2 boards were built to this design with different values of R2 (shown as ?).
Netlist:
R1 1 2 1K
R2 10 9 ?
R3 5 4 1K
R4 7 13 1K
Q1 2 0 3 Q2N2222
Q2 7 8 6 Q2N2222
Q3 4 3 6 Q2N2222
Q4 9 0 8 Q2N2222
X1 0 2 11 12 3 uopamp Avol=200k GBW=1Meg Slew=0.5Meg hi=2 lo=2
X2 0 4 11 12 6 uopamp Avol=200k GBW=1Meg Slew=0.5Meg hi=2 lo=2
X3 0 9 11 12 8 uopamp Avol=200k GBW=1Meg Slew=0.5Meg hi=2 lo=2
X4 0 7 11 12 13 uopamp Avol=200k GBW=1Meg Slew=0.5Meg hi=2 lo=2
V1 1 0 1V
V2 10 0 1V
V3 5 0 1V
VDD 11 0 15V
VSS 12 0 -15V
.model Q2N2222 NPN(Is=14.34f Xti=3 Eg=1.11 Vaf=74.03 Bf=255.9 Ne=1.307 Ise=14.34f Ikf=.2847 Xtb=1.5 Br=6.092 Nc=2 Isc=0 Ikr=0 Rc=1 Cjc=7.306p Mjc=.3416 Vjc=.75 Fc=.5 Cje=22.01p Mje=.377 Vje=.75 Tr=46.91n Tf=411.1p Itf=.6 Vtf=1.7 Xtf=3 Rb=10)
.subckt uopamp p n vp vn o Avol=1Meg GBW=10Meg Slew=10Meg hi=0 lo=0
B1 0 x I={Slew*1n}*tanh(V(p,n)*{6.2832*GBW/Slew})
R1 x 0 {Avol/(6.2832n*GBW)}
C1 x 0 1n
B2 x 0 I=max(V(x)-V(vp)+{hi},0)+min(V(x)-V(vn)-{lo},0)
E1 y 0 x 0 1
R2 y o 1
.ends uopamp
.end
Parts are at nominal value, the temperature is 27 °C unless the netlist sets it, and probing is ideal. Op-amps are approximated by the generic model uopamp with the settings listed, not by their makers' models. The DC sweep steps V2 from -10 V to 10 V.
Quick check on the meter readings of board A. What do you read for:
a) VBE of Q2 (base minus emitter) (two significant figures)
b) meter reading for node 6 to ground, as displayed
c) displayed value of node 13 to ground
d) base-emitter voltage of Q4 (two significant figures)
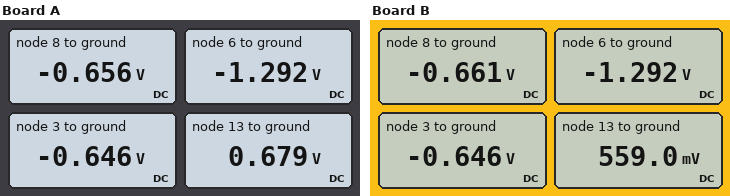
640 mV
-1.292 V
0.679 V
660 mV
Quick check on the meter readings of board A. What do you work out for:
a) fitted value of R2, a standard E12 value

680 Ω
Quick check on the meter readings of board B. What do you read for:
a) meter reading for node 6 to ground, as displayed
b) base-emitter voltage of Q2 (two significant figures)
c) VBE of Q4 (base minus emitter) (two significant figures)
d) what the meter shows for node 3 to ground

-1.292 V
630 mV
660 mV
-0.646 V
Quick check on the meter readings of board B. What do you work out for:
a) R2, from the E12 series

560 Ω
